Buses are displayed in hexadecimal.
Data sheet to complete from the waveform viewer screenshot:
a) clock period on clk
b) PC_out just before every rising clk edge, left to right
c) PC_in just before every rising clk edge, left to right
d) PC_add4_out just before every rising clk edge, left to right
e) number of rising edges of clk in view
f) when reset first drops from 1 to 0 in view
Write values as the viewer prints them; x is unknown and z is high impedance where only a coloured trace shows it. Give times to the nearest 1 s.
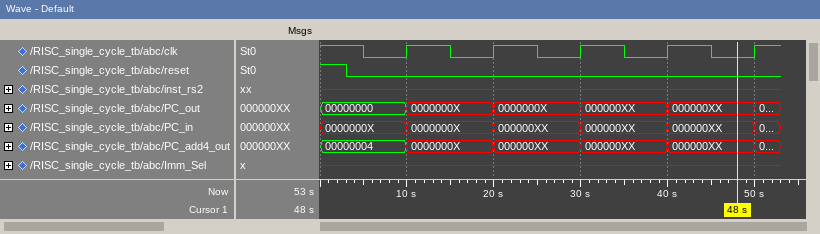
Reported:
10 s
00000000, 0000000X, 0000000X, 000000XX, 000000XX
0000000X, 0000000X, 000000XX, 000000XX, 000000XX
00000004, 0000000X, 000000XX, 000000XX, 000000XX
5
3 s
